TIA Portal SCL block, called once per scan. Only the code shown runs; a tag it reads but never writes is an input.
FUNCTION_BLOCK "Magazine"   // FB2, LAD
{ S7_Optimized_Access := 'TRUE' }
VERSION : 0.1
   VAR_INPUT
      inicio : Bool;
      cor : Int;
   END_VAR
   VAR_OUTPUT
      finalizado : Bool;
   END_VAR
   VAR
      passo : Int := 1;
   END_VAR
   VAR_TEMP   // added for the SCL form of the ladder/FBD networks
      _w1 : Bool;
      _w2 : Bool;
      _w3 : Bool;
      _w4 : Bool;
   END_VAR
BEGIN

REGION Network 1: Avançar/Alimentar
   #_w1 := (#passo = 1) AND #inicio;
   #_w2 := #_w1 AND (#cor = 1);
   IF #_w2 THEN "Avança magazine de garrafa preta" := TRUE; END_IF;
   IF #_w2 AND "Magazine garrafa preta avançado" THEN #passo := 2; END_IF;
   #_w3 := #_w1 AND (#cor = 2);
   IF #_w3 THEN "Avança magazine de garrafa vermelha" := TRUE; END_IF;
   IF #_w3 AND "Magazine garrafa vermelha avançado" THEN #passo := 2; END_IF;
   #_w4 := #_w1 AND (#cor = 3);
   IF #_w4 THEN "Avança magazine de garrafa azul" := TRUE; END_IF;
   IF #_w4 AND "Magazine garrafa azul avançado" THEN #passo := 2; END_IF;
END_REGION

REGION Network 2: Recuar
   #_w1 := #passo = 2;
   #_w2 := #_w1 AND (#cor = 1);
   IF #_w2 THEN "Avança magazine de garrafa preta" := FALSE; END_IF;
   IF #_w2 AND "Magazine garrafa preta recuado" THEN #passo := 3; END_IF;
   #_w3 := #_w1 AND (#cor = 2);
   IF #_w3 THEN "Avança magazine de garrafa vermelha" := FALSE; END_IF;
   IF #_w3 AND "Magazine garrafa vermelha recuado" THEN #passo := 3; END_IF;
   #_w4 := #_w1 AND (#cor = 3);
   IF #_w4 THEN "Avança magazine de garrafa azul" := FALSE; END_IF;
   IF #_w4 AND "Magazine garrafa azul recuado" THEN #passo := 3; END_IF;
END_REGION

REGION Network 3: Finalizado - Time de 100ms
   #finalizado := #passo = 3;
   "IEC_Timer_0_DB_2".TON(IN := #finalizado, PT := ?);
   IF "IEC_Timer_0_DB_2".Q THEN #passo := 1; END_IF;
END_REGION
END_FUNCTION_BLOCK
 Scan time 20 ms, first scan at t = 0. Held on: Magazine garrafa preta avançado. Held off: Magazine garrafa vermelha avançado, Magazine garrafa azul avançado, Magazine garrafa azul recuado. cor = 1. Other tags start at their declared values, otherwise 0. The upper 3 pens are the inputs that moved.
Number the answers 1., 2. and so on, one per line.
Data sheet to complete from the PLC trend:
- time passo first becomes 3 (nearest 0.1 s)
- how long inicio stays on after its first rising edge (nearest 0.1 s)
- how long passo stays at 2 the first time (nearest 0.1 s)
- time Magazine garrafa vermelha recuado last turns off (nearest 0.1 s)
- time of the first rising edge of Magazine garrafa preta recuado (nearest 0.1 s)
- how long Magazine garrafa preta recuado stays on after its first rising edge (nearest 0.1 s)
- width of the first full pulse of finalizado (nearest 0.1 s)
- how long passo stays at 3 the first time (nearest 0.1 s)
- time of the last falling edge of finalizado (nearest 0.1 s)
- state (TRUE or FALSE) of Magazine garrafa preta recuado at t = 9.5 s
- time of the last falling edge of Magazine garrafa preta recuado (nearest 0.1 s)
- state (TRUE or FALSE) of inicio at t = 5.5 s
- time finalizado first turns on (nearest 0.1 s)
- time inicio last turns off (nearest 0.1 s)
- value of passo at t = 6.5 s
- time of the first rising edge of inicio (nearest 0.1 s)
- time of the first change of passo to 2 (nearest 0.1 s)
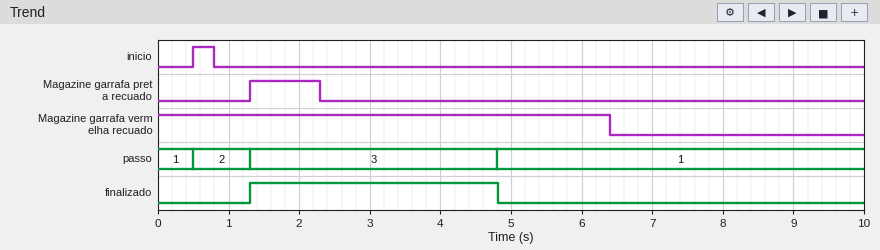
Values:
1. 1.3 s
2. 0.3 s
3. 0.8 s
4. 6.4 s
5. 1.3 s
6. 1.0 s
7. 3.5 s
8. 3.5 s
9. 4.8 s
10. FALSE
11. 2.3 s
12. FALSE
13. 1.3 s
14. 0.8 s
15. 1
16. 0.5 s
17. 0.5 s
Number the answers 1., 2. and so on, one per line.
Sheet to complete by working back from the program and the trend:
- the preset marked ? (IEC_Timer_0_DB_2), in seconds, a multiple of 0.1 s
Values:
1. 3.5 s
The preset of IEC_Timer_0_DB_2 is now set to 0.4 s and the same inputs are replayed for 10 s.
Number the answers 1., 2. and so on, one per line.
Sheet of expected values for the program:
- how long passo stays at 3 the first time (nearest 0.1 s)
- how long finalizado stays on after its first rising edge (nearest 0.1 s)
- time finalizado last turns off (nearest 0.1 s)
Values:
1. 0.4 s
2. 0.4 s
3. 1.7 s
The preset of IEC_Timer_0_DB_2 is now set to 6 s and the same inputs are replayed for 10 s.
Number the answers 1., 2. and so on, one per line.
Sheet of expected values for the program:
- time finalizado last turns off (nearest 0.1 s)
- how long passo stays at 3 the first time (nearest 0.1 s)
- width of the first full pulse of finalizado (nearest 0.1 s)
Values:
1. 7.3 s
2. 6.0 s
3. 6.0 s
